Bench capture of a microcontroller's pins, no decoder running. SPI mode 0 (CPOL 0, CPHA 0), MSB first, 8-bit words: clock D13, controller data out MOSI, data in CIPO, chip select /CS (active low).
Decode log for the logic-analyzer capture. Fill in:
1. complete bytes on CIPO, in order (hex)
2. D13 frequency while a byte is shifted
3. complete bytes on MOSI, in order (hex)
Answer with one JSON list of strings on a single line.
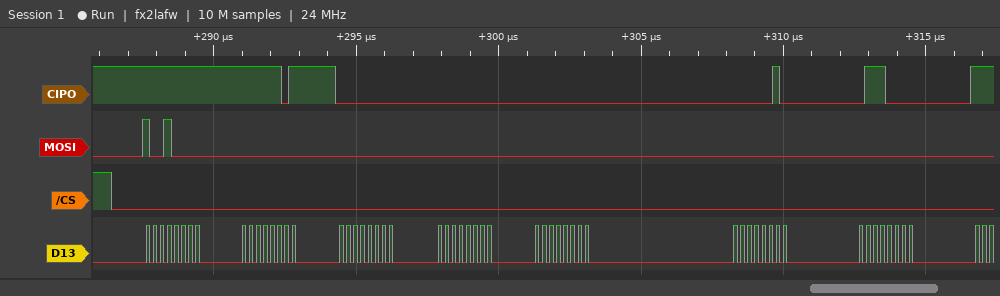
["FF FD 00 00 00 02 70", "4 MHz", "90 00 00 00 00 00 00"]
